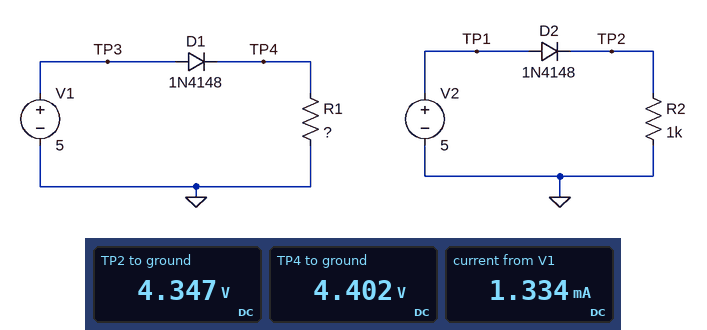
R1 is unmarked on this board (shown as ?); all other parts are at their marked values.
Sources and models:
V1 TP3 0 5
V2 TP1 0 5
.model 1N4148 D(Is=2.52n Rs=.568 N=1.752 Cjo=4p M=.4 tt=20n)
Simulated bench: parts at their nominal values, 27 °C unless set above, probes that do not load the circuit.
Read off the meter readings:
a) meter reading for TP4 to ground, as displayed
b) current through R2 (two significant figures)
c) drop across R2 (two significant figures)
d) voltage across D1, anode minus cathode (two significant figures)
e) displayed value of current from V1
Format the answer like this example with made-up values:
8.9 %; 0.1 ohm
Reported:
4.402 V; 4.3 mA; 4.3 V; 600 mV; 1.334 mA
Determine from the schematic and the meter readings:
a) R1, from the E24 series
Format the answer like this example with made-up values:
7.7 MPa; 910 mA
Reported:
3.3 kΩ
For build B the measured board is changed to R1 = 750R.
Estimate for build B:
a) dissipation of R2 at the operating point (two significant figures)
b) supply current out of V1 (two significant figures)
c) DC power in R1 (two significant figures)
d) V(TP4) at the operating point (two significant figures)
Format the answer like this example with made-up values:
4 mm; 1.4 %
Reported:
19 mW; 5.8 mA; 25 mW; 4.3 V
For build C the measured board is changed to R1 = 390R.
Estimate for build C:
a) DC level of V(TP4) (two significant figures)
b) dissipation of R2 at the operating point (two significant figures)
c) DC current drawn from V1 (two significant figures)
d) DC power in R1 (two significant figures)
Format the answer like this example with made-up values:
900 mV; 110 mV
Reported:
4.3 V; 19 mW; 11 mA; 47 mW
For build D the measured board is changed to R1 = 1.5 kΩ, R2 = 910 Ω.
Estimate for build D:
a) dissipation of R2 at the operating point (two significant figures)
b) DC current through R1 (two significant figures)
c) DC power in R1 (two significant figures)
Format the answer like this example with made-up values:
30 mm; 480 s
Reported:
21 mW; 2.9 mA; 13 mW
